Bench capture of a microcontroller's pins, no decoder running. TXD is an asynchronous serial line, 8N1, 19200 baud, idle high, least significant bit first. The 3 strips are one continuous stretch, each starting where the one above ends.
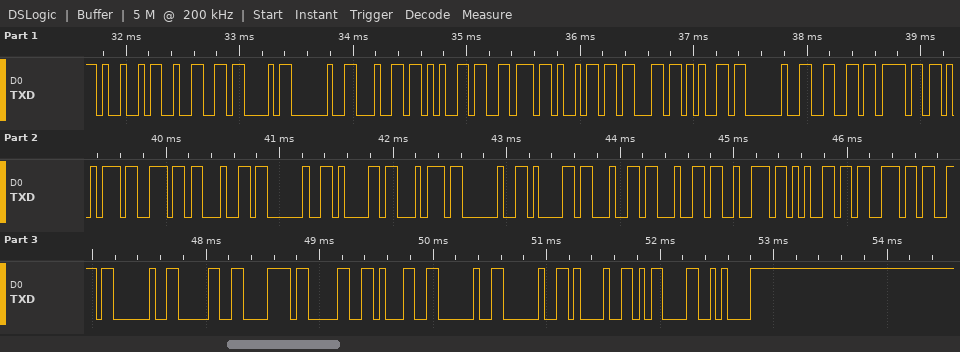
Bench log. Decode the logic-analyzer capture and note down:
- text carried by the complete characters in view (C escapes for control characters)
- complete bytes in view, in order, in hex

"I2C device found at address 0x01  !\r\n"
0x49 0x32 0x43 0x20 0x64 0x65 0x76 0x69 0x63 0x65 0x20 0x66 0x6F 0x75 0x6E 0x64 0x20 0x61 0x74 0x20 0x61 0x64 0x64 0x72 0x65 0x73 0x73 0x20 0x30 0x78 0x30 0x31 0x20 0x20 0x21 0x0D 0x0A
